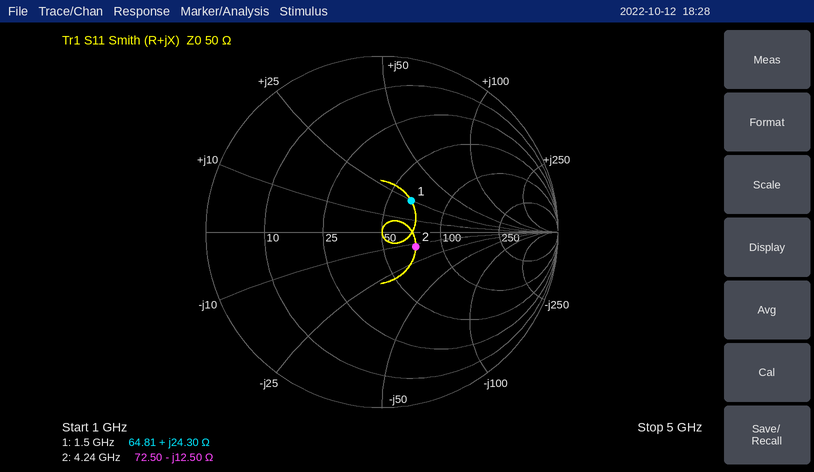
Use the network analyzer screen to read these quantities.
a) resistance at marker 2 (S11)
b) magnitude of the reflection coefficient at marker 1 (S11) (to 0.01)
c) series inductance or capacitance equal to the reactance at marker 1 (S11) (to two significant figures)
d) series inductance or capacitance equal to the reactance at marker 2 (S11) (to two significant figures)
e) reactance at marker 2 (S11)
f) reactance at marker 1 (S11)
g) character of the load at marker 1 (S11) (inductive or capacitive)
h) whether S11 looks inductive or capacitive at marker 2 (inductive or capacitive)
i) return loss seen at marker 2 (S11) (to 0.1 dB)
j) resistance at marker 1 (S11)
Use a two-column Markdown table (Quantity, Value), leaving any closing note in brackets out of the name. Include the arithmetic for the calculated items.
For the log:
| Quantity | Value |
|---|---|
| resistance at marker 2 | 72.50 Ω |
| magnitude of the reflection coefficient at marker 1 (S11) | 0.24 |
| series inductance or capacitance equal to the reactance at marker 1 (S11) | L = 24.3 Ω/(2π × 1.5 GHz) ≈ 2.6 nH |
| series inductance or capacitance equal to the reactance at marker 2 (S11) | C = 1/(2π × 4.24 GHz × 12.5 Ω) ≈ 3.0 pF |
| reactance at marker 2 | -12.50 Ω |
| reactance at marker 1 | +24.30 Ω |
| character of the load at marker 1 (S11) | inductive |
| whether S11 looks inductive or capacitive at marker 2 | capacitive |
| return loss seen at marker 2 (S11) | 13.6 dB |
| resistance at marker 1 | 64.81 Ω |
